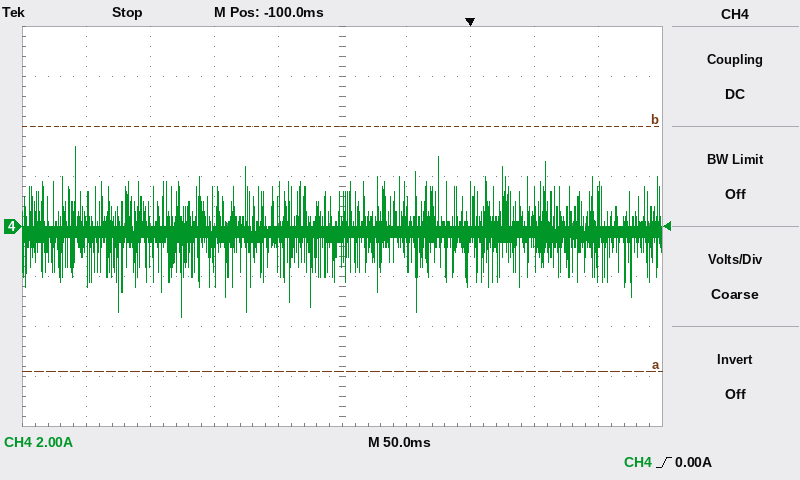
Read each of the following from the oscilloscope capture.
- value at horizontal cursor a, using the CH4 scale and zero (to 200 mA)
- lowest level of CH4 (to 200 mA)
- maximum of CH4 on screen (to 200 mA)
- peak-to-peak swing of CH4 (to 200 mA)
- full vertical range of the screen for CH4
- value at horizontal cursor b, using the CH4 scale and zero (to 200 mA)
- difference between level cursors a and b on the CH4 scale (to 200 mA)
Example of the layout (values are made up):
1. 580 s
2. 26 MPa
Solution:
1. -5.8 A
2. -3.6 A
3. 3.2 A
4. 6.8 A
5. 16 A
6. 4.0 A
7. 9.8 A
